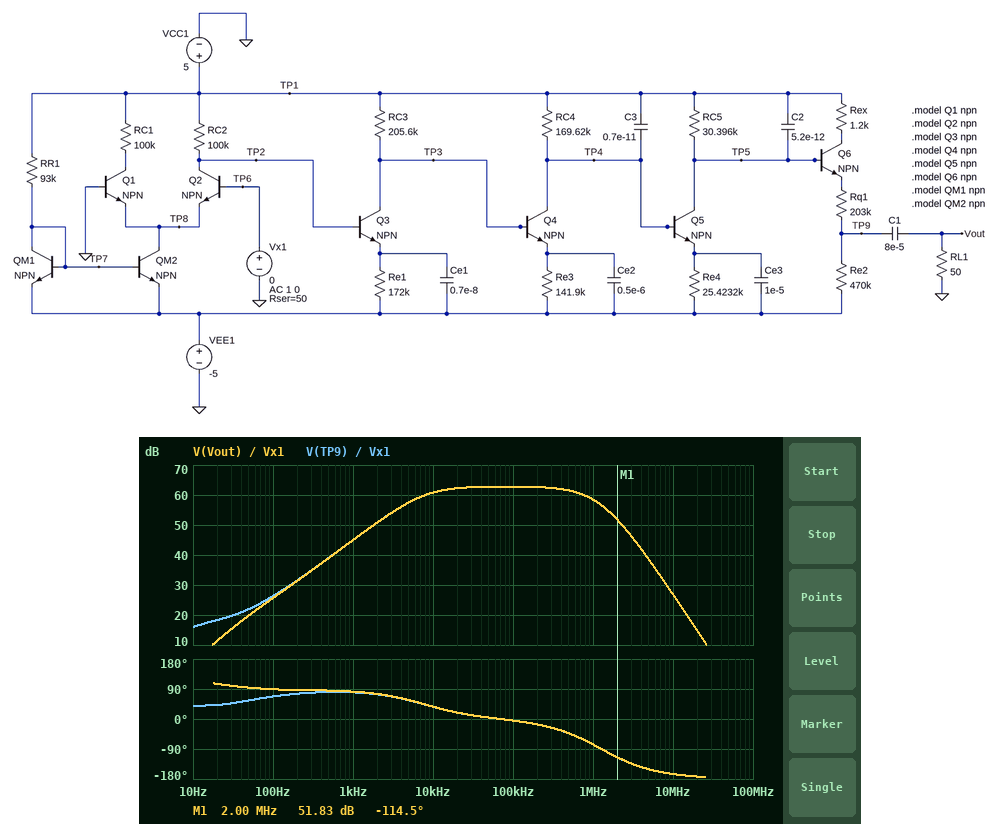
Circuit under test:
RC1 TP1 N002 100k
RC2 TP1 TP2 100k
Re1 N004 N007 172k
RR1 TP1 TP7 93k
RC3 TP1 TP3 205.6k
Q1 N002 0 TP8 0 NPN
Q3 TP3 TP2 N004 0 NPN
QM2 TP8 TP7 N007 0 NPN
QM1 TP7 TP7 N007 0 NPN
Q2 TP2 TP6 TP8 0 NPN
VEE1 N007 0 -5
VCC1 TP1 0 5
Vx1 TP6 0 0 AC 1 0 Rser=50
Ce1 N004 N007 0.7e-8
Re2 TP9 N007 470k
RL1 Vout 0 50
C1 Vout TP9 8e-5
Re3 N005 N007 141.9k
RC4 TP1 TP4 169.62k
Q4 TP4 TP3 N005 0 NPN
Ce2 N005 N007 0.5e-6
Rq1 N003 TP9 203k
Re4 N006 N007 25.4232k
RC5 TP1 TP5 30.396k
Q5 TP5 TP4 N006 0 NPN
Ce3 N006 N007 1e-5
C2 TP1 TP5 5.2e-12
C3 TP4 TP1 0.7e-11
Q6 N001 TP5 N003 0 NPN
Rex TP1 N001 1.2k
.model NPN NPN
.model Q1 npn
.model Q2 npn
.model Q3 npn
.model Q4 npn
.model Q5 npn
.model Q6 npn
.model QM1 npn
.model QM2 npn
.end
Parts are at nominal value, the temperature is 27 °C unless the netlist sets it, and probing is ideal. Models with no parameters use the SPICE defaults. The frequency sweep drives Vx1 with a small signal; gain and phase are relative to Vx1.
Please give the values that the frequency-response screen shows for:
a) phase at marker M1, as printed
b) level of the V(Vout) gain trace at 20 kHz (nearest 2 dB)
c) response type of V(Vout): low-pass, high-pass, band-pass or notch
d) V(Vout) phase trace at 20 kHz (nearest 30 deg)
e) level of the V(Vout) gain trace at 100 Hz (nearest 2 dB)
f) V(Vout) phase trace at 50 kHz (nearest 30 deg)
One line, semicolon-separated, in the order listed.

-114.5 deg; 62 dB; band-pass; 30 deg; 26 dB; 0 deg
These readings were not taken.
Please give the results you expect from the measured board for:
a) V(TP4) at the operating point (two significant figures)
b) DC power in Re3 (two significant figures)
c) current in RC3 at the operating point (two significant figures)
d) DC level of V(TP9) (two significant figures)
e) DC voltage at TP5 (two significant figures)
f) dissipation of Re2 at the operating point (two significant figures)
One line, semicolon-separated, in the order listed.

-9.1 mV; 110 µW; 26 µA; -2.0 V; -48 mV; 19 µW
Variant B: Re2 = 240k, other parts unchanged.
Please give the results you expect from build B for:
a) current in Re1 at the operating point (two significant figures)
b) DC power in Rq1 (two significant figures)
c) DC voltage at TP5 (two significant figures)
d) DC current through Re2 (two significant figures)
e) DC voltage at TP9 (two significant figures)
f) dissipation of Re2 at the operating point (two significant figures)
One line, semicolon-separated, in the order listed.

26 µA; 19 µW; -49 mV; 9.7 µA; -2.7 V; 23 µW
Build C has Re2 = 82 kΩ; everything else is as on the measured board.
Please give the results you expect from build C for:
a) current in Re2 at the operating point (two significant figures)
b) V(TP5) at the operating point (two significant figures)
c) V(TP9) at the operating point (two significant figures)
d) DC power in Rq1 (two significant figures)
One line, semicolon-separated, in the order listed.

15 µA; -51 mV; -3.8 V; 46 µW
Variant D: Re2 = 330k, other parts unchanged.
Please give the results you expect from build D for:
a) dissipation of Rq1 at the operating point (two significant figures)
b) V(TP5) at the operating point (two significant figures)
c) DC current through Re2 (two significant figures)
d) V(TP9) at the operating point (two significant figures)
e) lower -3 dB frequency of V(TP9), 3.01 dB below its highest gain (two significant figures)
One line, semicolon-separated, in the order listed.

13 µW; -49 mV; 8.1 µA; -2.3 V; 7.7 kHz
